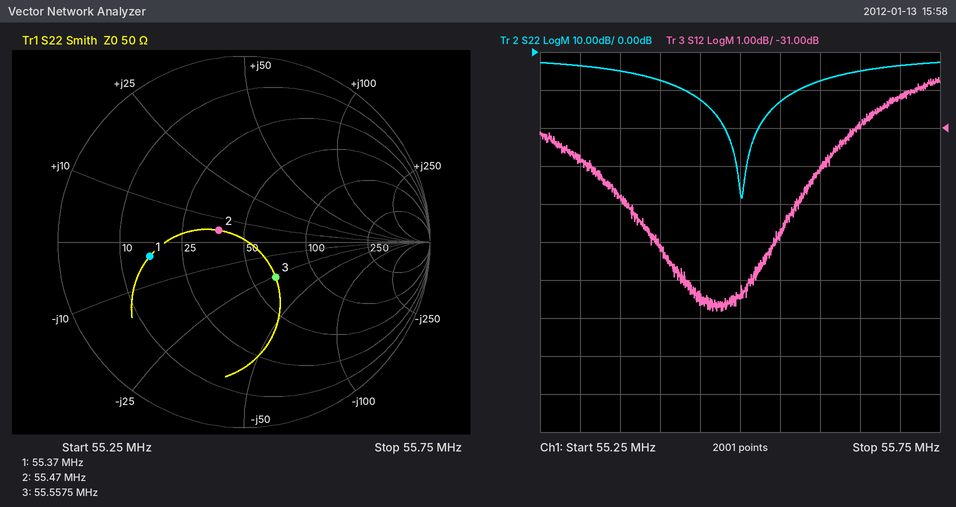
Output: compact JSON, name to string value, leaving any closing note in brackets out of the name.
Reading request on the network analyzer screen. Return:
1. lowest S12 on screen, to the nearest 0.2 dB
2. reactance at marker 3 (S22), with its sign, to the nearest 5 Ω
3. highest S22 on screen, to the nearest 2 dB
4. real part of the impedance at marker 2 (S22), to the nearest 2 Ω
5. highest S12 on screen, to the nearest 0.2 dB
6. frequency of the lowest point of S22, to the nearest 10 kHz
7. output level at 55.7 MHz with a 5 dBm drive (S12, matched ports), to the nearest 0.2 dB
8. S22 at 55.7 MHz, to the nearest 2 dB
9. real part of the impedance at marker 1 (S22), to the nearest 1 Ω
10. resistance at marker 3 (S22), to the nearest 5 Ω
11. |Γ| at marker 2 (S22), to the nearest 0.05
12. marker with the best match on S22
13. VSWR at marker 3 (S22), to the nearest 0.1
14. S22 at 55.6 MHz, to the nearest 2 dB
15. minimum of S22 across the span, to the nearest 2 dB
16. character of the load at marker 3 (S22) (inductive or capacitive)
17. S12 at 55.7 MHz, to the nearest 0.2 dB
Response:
{"lowest S12 on screen, to the nearest 0.2 dB": "-35.8 dB", "reactance at marker 3 (S22), with its sign, to the nearest 5 Ω": "-25 Ω", "highest S22 on screen, to the nearest 2 dB": "-2 dB", "real part of the impedance at marker 2 (S22), to the nearest 2 Ω": "38 Ω", "highest S12 on screen, to the nearest 0.2 dB": "-29.6 dB", "frequency of the lowest point of S22, to the nearest 10 kHz": "55.50 MHz", "output level at 55.7 MHz with a 5 dBm drive (S12, matched ports), to the nearest 0.2 dB": "-25.2 dBm", "S22 at 55.7 MHz, to the nearest 2 dB": "-4 dB", "real part of the impedance at marker 1 (S22), to the nearest 1 Ω": "16 Ω", "resistance at marker 3 (S22), to the nearest 5 Ω": "65 Ω", "|Γ| at marker 2 (S22), to the nearest 0.05": "0.15", "marker with the best match on S22": "marker 2", "VSWR at marker 3 (S22), to the nearest 0.1": "1.7", "S22 at 55.6 MHz, to the nearest 2 dB": "-8 dB", "minimum of S22 across the span, to the nearest 2 dB": "-38 dB", "character of the load at marker 3 (S22)": "capacitive", "S12 at 55.7 MHz, to the nearest 0.2 dB": "-30.2 dB"}
